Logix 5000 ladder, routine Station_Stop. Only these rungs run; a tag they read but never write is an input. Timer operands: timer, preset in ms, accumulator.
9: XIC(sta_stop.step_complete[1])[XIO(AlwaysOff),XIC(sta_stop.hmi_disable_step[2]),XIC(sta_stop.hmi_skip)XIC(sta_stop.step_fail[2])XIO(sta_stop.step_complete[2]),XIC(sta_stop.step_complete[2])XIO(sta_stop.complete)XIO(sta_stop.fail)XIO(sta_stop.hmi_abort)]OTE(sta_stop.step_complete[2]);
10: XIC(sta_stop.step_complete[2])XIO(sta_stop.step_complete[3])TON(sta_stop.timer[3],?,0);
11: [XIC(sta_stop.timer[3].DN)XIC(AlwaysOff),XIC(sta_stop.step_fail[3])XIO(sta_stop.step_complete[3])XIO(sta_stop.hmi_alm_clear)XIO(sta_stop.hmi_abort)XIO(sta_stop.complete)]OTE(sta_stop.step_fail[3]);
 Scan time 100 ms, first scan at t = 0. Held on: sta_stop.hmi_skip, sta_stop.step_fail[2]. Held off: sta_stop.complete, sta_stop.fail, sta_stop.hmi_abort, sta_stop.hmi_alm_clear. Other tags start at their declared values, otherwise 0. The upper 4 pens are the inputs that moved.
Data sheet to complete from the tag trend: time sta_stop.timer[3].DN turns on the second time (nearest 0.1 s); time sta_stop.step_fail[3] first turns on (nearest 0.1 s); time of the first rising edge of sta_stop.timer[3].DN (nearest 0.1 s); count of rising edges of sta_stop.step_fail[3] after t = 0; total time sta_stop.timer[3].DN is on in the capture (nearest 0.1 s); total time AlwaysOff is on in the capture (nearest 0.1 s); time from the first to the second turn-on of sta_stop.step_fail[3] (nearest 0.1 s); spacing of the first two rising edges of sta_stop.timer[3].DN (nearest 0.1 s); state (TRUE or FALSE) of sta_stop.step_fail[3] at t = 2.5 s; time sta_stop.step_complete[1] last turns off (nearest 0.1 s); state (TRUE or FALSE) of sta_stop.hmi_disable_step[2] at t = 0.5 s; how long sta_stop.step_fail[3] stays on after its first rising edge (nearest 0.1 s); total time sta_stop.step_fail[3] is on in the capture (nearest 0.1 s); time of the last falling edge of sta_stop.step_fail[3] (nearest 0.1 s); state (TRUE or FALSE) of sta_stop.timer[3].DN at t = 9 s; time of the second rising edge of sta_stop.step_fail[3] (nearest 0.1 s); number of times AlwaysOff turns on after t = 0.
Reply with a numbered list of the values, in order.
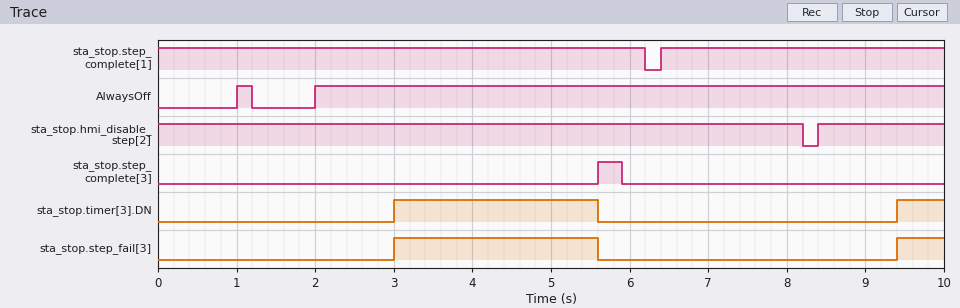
1. 9.4 s
2. 3.0 s
3. 3.0 s
4. 2
5. 3.2 s
6. 8.2 s
7. 6.4 s
8. 6.4 s
9. FALSE
10. 6.2 s
11. TRUE
12. 2.6 s
13. 3.2 s
14. 5.6 s
15. FALSE
16. 9.4 s
17. 2
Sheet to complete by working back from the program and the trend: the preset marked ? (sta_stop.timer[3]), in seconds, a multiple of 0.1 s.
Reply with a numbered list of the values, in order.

1. 3.0 s
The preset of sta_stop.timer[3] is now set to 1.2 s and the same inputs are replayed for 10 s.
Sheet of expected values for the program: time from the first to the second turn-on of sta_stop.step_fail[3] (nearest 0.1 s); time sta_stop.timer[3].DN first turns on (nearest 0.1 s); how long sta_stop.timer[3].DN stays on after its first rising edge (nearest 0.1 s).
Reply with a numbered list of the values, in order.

1. 5.6 s
2. 1.2 s
3. 4.4 s
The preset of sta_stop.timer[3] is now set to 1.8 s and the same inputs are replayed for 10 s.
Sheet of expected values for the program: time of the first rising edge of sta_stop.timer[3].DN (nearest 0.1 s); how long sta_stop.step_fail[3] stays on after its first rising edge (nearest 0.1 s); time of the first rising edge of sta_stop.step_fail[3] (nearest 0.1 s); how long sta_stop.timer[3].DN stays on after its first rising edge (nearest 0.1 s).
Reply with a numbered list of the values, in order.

1. 1.8 s
2. 3.6 s
3. 2.0 s
4. 3.8 s
